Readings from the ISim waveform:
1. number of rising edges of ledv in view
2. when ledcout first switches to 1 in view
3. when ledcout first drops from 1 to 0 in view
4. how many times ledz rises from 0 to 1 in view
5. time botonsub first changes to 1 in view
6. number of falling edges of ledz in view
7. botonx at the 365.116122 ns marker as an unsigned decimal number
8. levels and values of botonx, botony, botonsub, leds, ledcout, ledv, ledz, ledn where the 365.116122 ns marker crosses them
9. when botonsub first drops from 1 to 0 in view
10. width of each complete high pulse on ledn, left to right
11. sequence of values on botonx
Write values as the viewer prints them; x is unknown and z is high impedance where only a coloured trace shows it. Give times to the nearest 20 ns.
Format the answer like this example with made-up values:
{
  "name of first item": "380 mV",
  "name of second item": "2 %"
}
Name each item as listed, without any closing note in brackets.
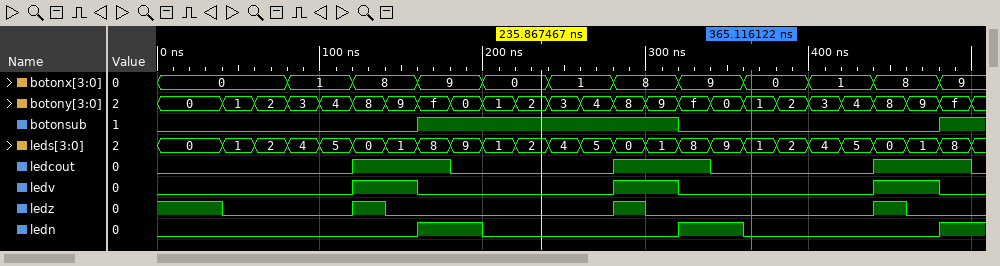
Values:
{
  "number of rising edges of ledv in view": "3",
  "when ledcout first switches to 1 in view": "120 ns",
  "when ledcout first drops from 1 to 0 in view": "180 ns",
  "how many times ledz rises from 0 to 1 in view": "3",
  "time botonsub first changes to 1 in view": "160 ns",
  "number of falling edges of ledz in view": "4",
  "botonx at the 365.116122 ns marker as an unsigned decimal number": "0",
  "levels and values of botonx, botony, botonsub, leds, ledcout, ledv, ledz, ledn where the 365.116122 ns marker crosses them": "botonx=0, botony=1, botonsub=0, leds=1, ledcout=0, ledv=0, ledz=0, ledn=0",
  "when botonsub first drops from 1 to 0 in view": "320 ns",
  "width of each complete high pulse on ledn, left to right": "40 ns, 40 ns",
  "sequence of values on botonx": "0, 1, 8, 9, 0, 1, 8, 9, 0, 1, 8, 9"
}
